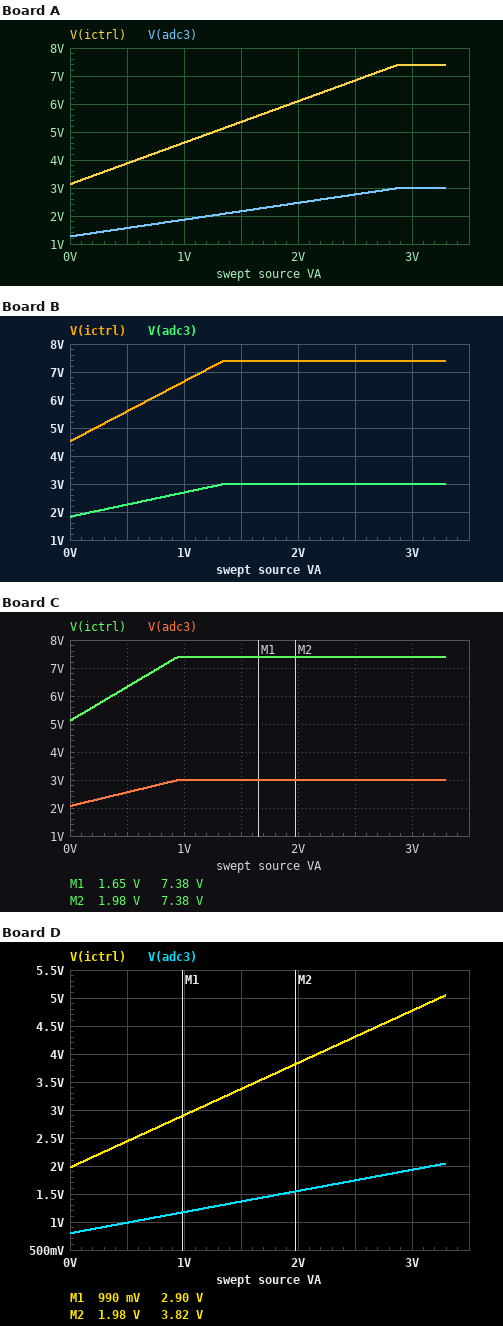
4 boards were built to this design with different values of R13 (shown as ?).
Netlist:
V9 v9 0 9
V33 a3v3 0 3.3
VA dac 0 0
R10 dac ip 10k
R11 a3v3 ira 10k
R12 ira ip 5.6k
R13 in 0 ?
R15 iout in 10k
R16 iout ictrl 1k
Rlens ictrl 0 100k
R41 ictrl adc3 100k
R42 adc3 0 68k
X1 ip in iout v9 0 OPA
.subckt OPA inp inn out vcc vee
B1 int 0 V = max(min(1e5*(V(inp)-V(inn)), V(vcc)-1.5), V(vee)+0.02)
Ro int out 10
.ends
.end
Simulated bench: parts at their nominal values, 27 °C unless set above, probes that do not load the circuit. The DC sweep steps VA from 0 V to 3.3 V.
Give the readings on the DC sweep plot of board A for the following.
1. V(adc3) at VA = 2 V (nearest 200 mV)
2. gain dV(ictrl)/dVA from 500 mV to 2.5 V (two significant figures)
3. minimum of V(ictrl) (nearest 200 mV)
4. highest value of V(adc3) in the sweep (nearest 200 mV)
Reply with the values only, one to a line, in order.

2.4 V
1.5 V/V
3.2 V
3.0 V
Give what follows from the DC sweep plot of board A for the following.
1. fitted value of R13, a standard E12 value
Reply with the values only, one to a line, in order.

6.8 kΩ
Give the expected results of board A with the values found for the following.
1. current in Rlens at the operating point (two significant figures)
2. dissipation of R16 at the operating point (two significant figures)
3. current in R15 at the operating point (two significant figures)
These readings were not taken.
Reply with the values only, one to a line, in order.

31 µA
2.5 µW
190 µA
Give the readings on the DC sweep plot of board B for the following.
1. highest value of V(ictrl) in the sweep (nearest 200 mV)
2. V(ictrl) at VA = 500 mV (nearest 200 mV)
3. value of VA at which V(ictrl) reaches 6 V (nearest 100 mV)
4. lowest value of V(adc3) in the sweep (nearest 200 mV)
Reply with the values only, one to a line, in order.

7.4 V
5.6 V
700 mV
1.8 V
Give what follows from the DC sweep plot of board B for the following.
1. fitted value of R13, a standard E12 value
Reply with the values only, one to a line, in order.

3.9 kΩ
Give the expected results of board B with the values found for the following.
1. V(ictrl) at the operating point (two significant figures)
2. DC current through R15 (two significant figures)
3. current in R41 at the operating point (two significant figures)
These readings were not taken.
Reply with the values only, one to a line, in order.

4.5 V
330 µA
27 µA
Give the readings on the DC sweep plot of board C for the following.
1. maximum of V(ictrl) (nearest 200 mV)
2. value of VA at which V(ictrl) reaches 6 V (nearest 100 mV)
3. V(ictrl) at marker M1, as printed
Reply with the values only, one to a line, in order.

7.4 V
400 mV
7.38 V
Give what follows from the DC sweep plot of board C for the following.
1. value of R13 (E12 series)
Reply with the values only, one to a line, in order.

3.3 kΩ
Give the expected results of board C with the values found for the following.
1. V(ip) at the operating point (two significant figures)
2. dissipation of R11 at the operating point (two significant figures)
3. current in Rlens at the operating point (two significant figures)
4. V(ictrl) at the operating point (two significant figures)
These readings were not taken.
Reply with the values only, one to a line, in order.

1.3 V
170 µW
51 µA
5.1 V
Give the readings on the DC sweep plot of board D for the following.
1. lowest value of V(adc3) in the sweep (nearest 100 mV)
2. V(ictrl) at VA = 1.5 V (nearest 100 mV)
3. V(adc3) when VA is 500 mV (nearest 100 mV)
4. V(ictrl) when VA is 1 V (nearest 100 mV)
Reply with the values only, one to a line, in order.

800 mV
3.4 V
1.0 V
2.9 V
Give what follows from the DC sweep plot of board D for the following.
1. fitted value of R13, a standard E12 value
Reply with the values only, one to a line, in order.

18 kΩ
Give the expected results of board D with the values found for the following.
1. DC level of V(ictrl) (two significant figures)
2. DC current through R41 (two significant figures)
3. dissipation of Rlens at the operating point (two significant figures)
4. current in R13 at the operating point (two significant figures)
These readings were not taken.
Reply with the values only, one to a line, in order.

2.0 V
12 µA
39 µW
72 µA
